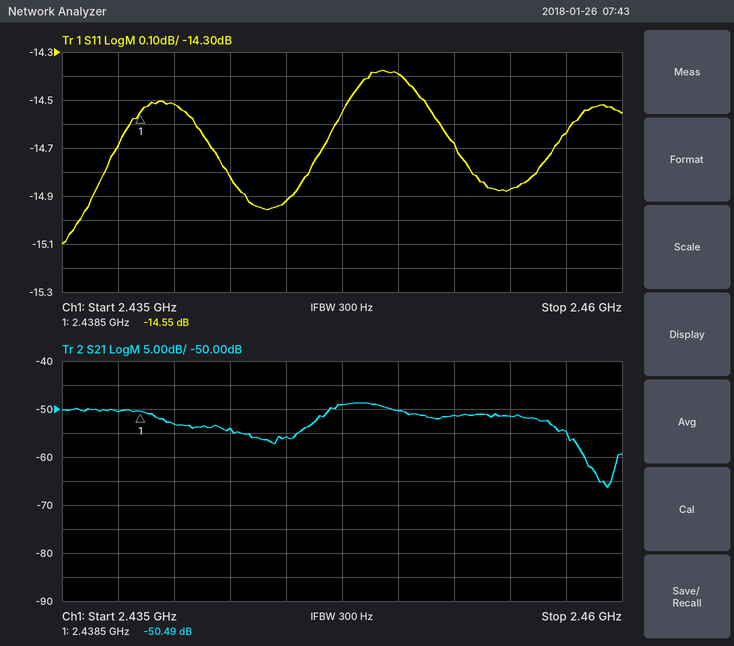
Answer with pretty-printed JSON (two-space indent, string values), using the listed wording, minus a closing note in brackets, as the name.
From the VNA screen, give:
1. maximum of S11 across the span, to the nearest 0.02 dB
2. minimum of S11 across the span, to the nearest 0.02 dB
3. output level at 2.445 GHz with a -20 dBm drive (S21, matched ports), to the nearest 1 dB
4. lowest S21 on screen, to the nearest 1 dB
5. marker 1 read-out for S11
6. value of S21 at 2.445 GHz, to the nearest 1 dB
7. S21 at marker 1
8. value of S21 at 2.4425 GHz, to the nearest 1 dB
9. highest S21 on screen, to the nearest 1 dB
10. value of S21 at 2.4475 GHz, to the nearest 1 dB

{
  "maximum of S11 across the span, to the nearest 0.02 dB": "-14.38 dB",
  "minimum of S11 across the span, to the nearest 0.02 dB": "-15.10 dB",
  "output level at 2.445 GHz with a -20 dBm drive (S21, matched ports), to the nearest 1 dB": "-76 dBm",
  "lowest S21 on screen, to the nearest 1 dB": "-66 dB",
  "marker 1 read-out for S11": "-14.55 dB",
  "value of S21 at 2.445 GHz, to the nearest 1 dB": "-56 dB",
  "S21 at marker 1": "-50.49 dB",
  "value of S21 at 2.4425 GHz, to the nearest 1 dB": "-54 dB",
  "highest S21 on screen, to the nearest 1 dB": "-49 dB",
  "value of S21 at 2.4475 GHz, to the nearest 1 dB": "-49 dB"
}
